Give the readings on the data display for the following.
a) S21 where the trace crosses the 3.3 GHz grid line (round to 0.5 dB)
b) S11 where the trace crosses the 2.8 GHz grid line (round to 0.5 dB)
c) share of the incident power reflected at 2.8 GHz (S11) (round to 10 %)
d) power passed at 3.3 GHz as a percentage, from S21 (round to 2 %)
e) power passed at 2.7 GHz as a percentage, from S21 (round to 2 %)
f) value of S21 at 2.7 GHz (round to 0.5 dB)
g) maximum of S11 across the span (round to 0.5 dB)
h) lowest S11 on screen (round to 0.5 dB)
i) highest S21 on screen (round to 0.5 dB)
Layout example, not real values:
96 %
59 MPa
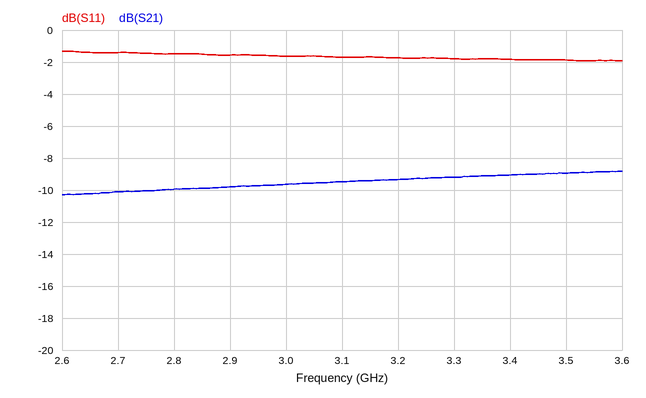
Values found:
-9.0 dB
-1.5 dB
70 %
12 %
10 %
-10.0 dB
-1.5 dB
-2.0 dB
-9.0 dB
